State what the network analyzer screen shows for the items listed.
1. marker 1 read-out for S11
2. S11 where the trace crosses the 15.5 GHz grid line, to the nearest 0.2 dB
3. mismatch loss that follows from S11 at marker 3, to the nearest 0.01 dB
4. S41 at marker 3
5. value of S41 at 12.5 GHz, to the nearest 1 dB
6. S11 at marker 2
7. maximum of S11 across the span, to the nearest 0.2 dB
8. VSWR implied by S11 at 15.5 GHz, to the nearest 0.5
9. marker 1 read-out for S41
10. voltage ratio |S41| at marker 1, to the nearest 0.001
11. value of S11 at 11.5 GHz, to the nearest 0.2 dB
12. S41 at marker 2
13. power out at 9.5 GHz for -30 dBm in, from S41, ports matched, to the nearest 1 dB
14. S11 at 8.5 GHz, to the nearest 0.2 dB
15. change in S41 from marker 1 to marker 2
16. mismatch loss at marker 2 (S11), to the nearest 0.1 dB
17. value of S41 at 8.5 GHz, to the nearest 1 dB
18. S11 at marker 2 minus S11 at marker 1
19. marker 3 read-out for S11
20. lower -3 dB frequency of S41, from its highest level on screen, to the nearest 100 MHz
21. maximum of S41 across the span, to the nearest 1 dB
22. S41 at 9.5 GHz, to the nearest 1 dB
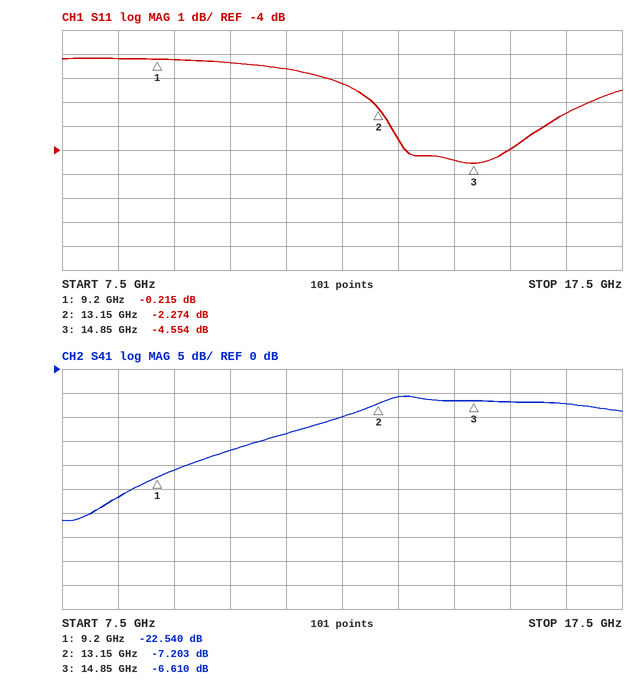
-0.215 dB
-4.0 dB
1.87 dB
-6.610 dB
-10 dB
-2.274 dB
-0.2 dB
4.5
-22.540 dB
0.075
-0.6 dB
-7.203 dB
-51 dBm
-0.2 dB
15.337 dB
3.9 dB
-27 dB
-2.059 dB
-4.554 dB
12.8 GHz
-6 dB
-21 dB
